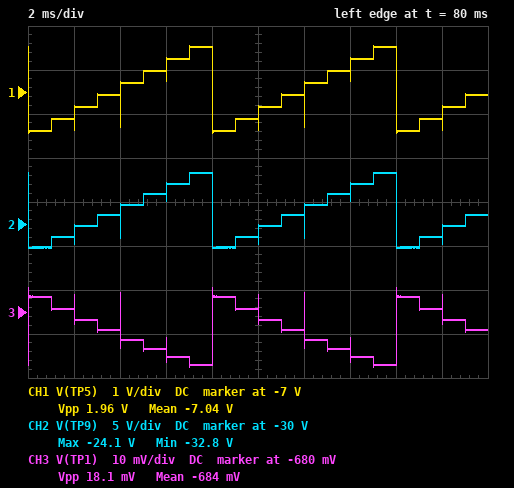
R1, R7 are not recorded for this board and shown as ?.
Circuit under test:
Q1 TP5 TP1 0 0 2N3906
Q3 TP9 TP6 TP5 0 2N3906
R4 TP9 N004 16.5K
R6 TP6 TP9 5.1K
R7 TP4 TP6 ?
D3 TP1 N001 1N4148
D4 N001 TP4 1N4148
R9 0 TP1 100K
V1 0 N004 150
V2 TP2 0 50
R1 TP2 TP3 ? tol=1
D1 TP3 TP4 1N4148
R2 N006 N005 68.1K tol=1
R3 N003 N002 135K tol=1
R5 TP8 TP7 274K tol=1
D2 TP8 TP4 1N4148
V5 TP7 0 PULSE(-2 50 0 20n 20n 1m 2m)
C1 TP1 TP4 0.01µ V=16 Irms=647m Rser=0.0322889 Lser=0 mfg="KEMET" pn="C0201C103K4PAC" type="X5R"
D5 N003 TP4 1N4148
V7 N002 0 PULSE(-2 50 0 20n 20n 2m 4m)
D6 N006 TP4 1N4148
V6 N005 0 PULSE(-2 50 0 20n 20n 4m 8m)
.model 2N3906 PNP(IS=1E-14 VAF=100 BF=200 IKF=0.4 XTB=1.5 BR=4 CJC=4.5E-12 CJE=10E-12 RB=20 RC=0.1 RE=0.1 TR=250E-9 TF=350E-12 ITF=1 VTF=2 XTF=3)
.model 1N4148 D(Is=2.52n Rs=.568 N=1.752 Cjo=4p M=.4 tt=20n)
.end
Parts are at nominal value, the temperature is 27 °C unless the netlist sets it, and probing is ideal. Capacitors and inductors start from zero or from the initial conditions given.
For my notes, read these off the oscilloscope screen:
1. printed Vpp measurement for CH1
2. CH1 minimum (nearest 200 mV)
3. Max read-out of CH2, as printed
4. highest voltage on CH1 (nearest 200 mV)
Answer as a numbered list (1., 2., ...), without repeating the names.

1. 1.96 V
2. -8.0 V
3. -24.1 V
4. -6.0 V
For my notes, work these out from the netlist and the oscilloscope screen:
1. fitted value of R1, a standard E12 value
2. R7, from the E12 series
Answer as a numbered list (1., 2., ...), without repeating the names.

1. 15 kΩ
2. 1.5 kΩ
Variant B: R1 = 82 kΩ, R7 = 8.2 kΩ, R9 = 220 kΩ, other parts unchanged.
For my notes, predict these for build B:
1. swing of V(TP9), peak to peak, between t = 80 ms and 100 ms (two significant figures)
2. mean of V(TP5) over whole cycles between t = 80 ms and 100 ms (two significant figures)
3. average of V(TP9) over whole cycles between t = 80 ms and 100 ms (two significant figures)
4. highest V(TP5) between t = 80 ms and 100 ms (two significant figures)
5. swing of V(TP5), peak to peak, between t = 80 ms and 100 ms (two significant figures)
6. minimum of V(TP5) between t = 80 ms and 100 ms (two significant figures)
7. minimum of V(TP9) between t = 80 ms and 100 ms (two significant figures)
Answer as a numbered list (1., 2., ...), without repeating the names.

1. 17 V
2. -12 V
3. -19 V
4. -6.3 V
5. 11 V
6. -17 V
7. -28 V
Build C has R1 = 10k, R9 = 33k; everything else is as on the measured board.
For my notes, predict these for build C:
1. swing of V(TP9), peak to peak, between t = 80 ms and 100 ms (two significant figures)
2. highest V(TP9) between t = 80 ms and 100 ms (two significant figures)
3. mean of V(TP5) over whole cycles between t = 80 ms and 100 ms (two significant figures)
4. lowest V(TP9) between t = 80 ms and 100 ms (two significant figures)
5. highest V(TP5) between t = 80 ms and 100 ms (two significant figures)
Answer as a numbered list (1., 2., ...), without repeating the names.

1. 8.4 V
2. -35 V
3. -9.5 V
4. -44 V
5. -8.5 V
